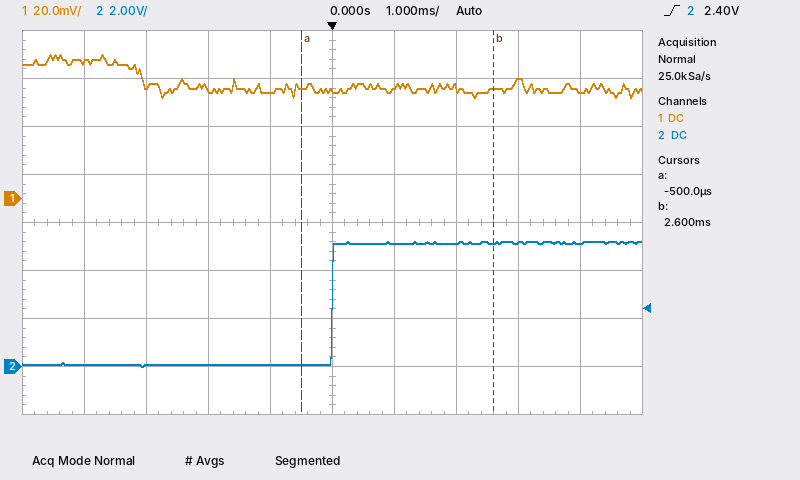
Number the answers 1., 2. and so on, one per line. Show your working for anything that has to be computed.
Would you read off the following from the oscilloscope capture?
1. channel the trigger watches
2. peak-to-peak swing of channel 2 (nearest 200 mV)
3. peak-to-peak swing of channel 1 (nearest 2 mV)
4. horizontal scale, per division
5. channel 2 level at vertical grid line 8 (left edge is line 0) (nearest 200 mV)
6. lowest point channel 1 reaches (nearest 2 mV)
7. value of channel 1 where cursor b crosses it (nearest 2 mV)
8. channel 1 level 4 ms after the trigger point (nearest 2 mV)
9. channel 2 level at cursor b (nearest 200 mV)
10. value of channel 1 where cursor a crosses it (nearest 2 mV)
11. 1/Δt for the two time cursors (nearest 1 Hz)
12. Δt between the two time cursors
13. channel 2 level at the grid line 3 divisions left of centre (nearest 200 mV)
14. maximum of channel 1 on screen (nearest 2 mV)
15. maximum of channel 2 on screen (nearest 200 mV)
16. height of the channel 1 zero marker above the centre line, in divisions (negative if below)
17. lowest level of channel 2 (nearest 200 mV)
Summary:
1. channel 2
2. 5.2 V − (0.0 V) = 5.2 V
3. 60 mV − (42 mV) = 18 mV
4. 1 ms
5. 5.2 V
6. 42 mV
7. 46 mV
8. 44 mV
9. 5.2 V
10. 46 mV
11. 1 / 3.1 ms ≈ 323 Hz
12. 2.6 ms − (-500 µs) = 3.1 ms
13. 0.0 V
14. 60 mV
15. 5.2 V
16. +0.5 div
17. 0.0 V
